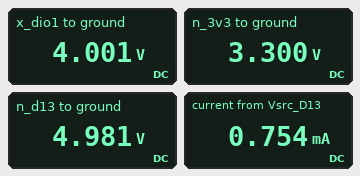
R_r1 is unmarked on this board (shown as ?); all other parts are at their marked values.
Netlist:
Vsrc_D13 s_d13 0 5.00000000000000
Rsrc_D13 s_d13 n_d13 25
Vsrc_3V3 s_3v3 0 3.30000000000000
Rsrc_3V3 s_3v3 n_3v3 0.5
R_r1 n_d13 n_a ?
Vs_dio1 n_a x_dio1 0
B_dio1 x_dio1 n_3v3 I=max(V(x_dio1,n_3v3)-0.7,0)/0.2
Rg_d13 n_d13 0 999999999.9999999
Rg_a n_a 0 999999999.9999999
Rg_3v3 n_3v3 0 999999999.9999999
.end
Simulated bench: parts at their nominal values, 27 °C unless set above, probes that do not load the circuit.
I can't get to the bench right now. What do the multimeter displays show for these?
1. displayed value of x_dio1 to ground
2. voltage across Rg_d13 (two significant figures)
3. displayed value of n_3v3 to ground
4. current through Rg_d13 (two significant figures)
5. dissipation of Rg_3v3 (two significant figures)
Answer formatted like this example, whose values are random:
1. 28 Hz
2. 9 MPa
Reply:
1. 4.001 V
2. 5.0 V
3. 3.300 V
4. 5.0 nA
5. 11 nW
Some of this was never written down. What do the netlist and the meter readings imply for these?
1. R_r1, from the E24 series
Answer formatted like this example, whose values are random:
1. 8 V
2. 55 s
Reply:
1. 1.3 kΩ
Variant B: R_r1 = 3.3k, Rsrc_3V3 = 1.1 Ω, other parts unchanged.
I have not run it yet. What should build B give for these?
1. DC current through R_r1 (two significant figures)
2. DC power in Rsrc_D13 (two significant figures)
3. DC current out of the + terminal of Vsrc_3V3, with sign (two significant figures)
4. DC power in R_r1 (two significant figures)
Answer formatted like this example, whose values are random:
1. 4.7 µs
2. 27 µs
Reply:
1. 300 µA
2. 2.3 µW
3. -300 µA
4. 300 µW
